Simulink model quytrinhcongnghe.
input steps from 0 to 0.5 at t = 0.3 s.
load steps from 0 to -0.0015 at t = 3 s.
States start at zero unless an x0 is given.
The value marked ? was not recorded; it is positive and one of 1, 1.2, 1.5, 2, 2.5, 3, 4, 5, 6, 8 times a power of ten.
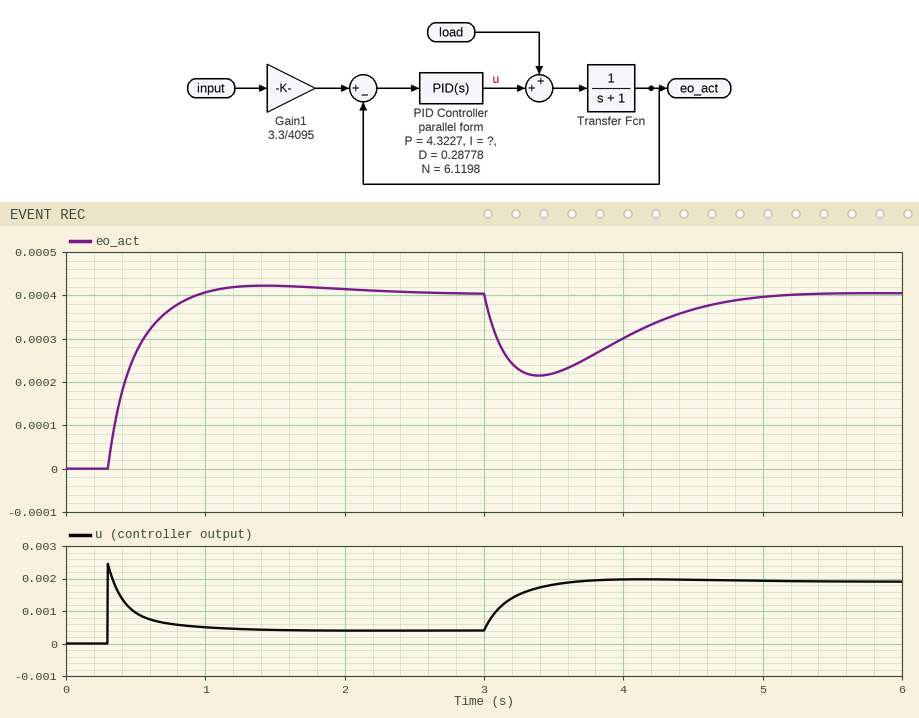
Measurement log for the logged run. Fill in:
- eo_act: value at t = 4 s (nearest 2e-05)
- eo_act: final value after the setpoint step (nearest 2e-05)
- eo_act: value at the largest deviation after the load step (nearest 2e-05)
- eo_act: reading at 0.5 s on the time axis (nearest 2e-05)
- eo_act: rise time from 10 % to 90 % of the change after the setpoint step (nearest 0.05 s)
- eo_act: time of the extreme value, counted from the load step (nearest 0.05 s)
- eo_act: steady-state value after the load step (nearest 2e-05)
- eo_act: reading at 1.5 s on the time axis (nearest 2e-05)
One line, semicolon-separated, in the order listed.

0.00030; 0.00040; 0.00022; 0.00026; 0.40 s; 0.40 s; 0.00040; 0.00042
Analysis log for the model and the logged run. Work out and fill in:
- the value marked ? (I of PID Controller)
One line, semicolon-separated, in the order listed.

8
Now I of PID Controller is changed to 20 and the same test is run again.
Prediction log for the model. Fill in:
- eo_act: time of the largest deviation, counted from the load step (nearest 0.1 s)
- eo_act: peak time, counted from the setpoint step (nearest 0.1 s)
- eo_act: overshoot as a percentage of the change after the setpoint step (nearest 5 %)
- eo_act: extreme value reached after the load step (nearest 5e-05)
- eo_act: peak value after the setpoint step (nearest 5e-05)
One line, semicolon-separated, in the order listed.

0.3 s; 0.6 s; 15 %; 0.00025; 0.00045
